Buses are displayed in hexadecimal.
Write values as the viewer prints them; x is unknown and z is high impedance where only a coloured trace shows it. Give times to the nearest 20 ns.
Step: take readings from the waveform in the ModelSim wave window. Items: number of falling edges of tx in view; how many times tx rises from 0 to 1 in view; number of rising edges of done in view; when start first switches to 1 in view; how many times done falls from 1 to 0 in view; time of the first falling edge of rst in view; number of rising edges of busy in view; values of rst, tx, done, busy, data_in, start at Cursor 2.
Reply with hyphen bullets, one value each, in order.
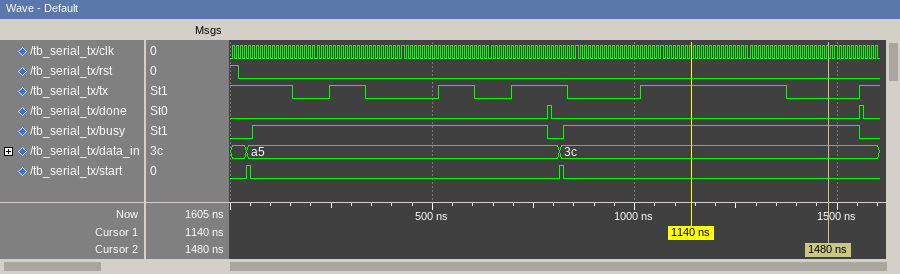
- 5
- 5
- 2
- 40 ns
- 2
- 20 ns
- 2
- rst=0, tx=0, done=0, busy=1, data_in=3c, start=0
